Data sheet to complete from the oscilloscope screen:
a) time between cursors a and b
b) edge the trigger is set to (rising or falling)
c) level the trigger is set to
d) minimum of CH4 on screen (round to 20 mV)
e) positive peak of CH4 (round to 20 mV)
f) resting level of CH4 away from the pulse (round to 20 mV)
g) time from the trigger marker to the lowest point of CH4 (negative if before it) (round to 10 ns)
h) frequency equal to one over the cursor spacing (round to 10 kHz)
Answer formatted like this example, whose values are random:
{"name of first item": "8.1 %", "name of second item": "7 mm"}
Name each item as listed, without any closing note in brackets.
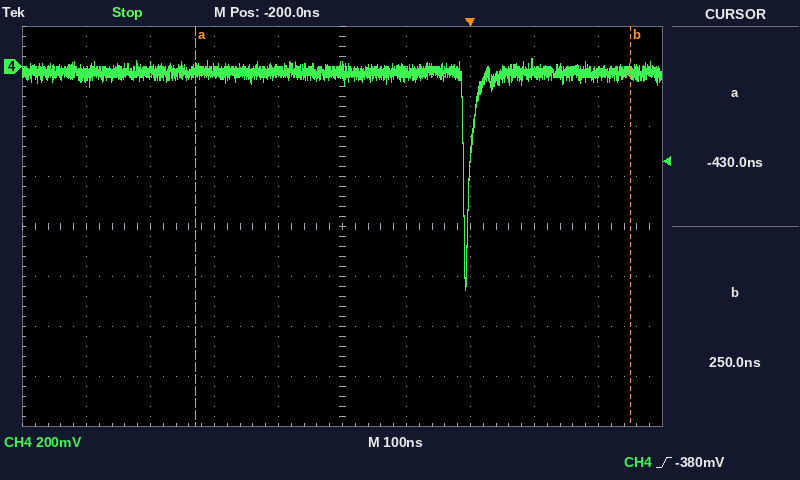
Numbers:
{"time between cursors a and b": "680 ns", "edge the trigger is set to": "rising", "level the trigger is set to": "-380 mV", "minimum of CH4 on screen": "-900 mV", "positive peak of CH4": "40 mV", "resting level of CH4 away from the pulse": "-20 mV", "time from the trigger marker to the lowest point of CH4 (negative if before it)": "-10 ns", "frequency equal to one over the cursor spacing": "1.47 MHz"}
